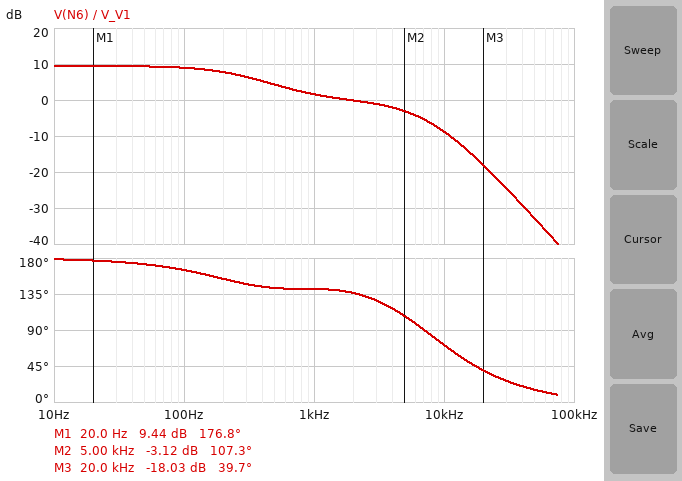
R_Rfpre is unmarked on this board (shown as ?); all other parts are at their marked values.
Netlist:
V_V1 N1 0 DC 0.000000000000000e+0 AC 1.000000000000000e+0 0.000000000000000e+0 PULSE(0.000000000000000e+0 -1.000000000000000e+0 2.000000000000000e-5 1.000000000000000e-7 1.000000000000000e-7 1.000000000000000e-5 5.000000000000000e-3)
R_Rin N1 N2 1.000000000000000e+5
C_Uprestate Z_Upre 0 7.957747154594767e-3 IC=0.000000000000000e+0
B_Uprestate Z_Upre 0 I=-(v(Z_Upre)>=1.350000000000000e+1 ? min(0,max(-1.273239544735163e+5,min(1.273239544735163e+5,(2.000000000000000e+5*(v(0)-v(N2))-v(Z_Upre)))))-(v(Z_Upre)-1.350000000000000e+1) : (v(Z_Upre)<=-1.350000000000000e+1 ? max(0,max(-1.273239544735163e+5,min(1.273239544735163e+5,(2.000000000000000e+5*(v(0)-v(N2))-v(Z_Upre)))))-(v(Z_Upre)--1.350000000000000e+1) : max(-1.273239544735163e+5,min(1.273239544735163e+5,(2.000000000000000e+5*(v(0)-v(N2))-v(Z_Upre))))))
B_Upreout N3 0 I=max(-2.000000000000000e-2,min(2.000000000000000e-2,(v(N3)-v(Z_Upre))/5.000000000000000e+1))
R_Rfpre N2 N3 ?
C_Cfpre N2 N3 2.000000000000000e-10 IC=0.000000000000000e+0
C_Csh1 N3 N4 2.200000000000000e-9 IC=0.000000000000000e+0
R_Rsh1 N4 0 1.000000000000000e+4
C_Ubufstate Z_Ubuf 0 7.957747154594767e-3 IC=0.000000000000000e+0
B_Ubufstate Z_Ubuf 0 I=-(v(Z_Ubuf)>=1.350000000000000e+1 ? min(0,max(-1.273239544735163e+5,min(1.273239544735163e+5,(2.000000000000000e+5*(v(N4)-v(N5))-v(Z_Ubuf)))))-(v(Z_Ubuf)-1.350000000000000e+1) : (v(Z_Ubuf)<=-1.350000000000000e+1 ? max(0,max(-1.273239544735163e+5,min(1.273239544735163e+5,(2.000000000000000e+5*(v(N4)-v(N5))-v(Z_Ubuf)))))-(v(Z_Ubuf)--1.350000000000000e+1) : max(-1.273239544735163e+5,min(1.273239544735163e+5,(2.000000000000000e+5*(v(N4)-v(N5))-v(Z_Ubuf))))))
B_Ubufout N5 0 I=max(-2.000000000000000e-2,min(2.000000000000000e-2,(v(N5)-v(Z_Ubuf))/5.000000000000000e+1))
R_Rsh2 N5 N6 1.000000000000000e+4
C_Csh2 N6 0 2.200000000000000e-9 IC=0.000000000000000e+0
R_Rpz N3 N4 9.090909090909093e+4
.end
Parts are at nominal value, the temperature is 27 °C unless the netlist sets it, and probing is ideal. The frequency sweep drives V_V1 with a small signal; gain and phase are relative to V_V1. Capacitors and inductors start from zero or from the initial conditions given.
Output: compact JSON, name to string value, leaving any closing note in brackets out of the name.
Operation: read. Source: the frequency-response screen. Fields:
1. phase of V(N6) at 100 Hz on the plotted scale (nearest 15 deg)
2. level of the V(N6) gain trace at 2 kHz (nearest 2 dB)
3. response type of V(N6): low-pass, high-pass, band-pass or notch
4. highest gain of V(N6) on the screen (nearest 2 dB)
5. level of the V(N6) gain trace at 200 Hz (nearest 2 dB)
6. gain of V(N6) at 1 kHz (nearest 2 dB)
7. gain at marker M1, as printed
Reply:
{"phase of V(N6) at 100 Hz on the plotted scale": "165 deg", "level of the V(N6) gain trace at 2 kHz": "0 dB", "response type of V(N6): low-pass, high-pass, band-pass or notch": "low-pass", "highest gain of V(N6) on the screen": "10 dB", "level of the V(N6) gain trace at 200 Hz": "8 dB", "gain of V(N6) at 1 kHz": "2 dB", "gain at marker M1, as printed": "9.44 dB"}
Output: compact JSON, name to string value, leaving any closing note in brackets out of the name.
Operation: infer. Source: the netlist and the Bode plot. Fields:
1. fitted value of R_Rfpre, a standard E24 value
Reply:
{"fitted value of R_Rfpre, a standard E24 value": "3 MΩ"}
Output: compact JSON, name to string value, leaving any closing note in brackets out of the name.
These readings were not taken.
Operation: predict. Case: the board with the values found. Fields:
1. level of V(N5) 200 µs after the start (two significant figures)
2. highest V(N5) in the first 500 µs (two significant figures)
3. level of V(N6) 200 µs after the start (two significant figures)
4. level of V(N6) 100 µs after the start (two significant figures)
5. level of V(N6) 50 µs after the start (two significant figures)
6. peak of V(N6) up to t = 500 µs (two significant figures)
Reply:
{"level of V(N5) 200 µs after the start": "26 mV", "highest V(N5) in the first 500 µs": "400 mV", "level of V(N6) 200 µs after the start": "28 mV", "level of V(N6) 100 µs after the start": "75 mV", "level of V(N6) 50 µs after the start": "180 mV", "peak of V(N6) up to t = 500 µs": "180 mV"}
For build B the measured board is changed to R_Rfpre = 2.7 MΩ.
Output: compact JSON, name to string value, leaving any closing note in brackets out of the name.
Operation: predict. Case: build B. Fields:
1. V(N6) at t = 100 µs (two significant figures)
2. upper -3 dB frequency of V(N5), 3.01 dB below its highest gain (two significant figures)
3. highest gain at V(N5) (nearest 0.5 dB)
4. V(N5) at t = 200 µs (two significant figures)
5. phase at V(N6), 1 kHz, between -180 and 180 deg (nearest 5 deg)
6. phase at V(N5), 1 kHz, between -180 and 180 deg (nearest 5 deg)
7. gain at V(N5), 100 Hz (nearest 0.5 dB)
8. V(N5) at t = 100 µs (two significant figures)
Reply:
{"V(N6) at t = 100 µs": "73 mV", "upper -3 dB frequency of V(N5), 3.01 dB below its highest gain": "340 Hz", "highest gain at V(N5)": "8.5 dB", "V(N5) at t = 200 µs": "24 mV", "phase at V(N6), 1 kHz, between -180 and 180 deg": "145 deg", "phase at V(N5), 1 kHz, between -180 and 180 deg": "150 deg", "gain at V(N5), 100 Hz": "8.0 dB", "V(N5) at t = 100 µs": "39 mV"}
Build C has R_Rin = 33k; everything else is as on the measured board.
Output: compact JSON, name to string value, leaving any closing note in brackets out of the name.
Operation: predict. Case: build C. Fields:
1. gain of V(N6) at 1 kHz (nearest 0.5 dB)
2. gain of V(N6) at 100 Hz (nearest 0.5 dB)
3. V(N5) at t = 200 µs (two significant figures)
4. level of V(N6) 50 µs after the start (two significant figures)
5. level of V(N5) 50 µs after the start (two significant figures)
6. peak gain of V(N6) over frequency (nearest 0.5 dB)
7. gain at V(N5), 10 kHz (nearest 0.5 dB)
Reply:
{"gain of V(N6) at 1 kHz": "11.0 dB", "gain of V(N6) at 100 Hz": "18.5 dB", "V(N5) at t = 200 µs": "78 mV", "level of V(N6) 50 µs after the start": "550 mV", "level of V(N5) 50 µs after the start": "510 mV", "peak gain of V(N6) over frequency": "19.0 dB", "gain at V(N5), 10 kHz": "5.5 dB"}
